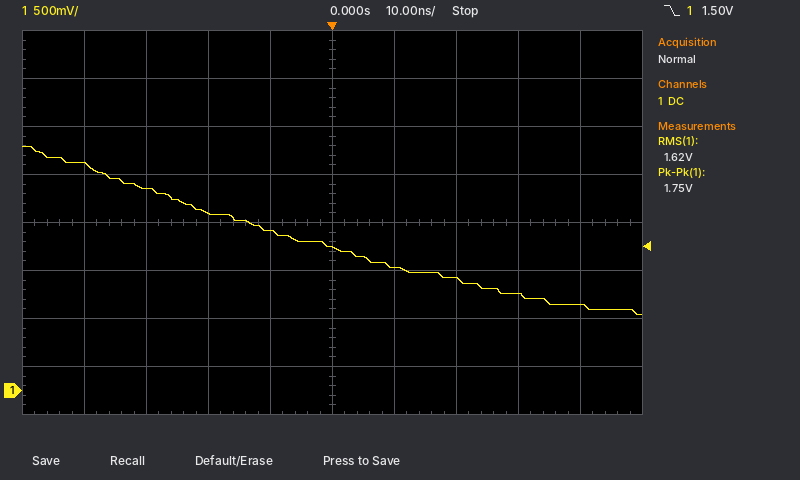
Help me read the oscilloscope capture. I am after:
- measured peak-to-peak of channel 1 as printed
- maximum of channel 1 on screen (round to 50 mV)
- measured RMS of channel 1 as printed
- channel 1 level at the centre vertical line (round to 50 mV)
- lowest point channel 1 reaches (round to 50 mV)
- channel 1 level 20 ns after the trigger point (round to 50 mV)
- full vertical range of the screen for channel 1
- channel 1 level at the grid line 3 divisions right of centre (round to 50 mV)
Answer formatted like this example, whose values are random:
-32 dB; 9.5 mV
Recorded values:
1.75 V; 2.55 V; 1.62 V; 1.50 V; 800 mV; 1.15 V; 4 V; 1.00 V
